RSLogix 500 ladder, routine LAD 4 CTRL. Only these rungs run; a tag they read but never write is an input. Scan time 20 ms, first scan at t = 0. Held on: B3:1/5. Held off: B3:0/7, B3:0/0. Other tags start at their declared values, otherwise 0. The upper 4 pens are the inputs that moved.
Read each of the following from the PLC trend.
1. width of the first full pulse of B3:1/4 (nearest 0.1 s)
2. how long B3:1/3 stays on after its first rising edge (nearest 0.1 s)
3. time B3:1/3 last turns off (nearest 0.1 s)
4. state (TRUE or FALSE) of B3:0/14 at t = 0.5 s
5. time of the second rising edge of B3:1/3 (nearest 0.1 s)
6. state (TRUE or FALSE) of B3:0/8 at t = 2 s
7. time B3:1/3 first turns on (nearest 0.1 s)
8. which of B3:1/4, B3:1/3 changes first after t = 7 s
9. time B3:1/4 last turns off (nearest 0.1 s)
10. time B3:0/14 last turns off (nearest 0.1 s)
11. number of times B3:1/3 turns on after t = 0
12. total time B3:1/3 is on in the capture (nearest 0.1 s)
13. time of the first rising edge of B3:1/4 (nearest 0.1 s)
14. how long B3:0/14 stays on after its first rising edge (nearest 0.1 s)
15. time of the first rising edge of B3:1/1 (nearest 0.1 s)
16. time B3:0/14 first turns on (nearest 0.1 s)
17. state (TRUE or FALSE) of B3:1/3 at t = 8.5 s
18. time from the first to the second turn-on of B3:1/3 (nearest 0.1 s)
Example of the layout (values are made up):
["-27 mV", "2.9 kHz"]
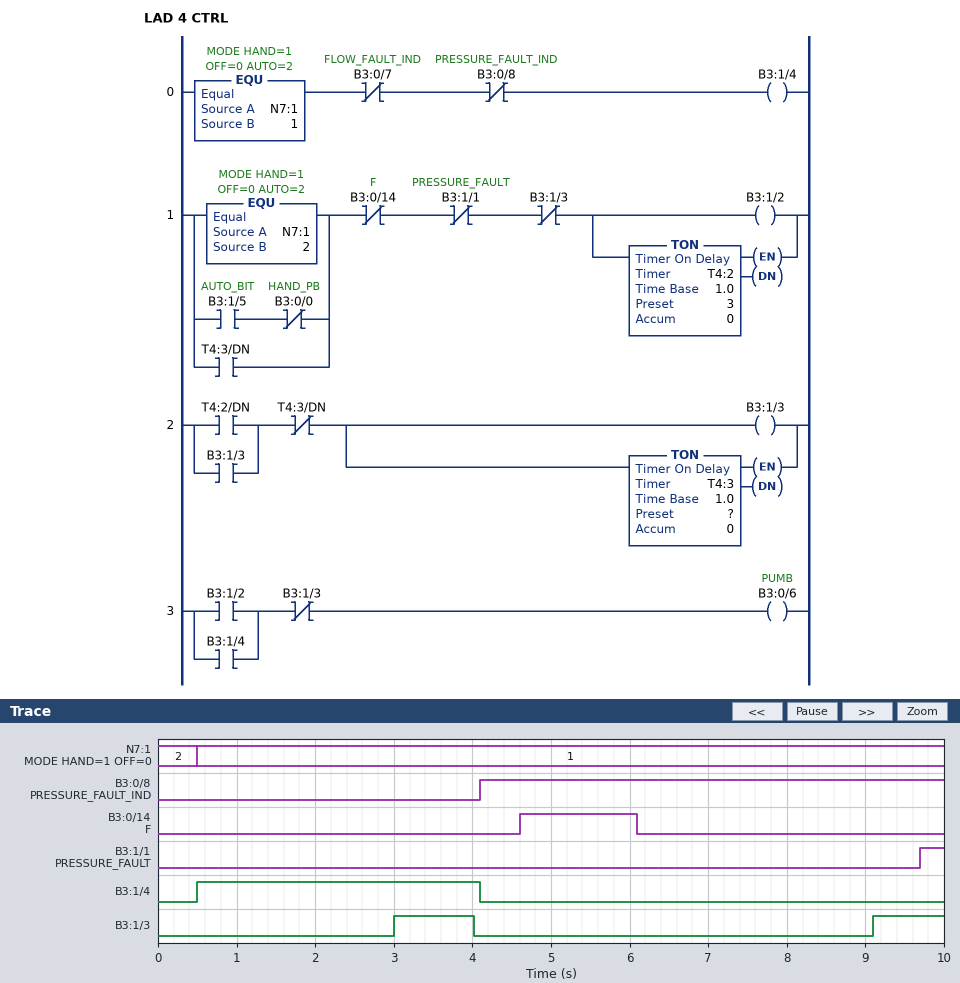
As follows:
["3.6 s", "1.0 s", "4.0 s", "FALSE", "9.1 s", "FALSE", "3.0 s", "B3:1/3", "4.1 s", "6.1 s", "2", "1.9 s", "0.5 s", "1.5 s", "9.7 s", "4.6 s", "FALSE", "6.1 s"]
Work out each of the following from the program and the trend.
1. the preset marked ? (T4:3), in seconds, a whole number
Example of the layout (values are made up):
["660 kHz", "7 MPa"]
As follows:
["1 s"]
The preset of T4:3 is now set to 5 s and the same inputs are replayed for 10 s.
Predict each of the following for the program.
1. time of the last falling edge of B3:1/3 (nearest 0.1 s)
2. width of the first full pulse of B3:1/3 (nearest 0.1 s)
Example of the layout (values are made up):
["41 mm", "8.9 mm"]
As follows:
["8.0 s", "5.0 s"]
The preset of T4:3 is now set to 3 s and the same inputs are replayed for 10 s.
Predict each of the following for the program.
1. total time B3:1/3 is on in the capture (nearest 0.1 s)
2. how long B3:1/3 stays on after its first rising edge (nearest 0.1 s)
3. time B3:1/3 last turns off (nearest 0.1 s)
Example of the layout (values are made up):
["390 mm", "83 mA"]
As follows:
["3.9 s", "3.0 s", "6.0 s"]
